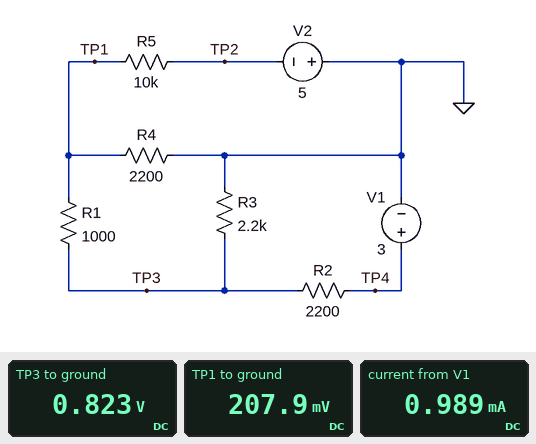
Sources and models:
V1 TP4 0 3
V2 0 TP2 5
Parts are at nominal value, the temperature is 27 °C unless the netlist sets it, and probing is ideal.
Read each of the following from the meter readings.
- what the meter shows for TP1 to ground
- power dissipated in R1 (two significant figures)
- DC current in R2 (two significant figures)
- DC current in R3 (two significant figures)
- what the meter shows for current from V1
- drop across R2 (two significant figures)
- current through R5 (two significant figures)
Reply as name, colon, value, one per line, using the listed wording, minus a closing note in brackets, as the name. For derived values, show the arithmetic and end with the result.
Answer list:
what the meter shows for TP1 to ground: 207.9 mV
power dissipated in R1: (823 mV - 207.9 mV)^2 / 1 kΩ = 380 µW
DC current in R2: (3 V - 823 mV) / 2.2 kΩ = 990 µA
DC current in R3: (823 mV) / 2.2 kΩ = 370 µA
what the meter shows for current from V1: 0.989 mA
drop across R2: 3 V - 823 mV = 2.2 V
current through R5: (207.9 mV - (-5 V)) / 10 kΩ = 520 µA
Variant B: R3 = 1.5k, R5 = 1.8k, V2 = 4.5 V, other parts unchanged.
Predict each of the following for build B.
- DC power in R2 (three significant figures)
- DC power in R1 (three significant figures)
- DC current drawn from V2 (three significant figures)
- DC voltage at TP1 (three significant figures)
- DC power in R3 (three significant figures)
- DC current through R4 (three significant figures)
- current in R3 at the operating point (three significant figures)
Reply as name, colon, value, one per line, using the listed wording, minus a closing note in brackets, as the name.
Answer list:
DC power in R2: 3.89 mW
DC power in R1: 1.64 mW
DC current drawn from V2: 1.83 mA
DC voltage at TP1: -1.21 V
DC power in R3: 3.64 µW
DC current through R4: 549 µA
current in R3 at the operating point: 49.2 µA
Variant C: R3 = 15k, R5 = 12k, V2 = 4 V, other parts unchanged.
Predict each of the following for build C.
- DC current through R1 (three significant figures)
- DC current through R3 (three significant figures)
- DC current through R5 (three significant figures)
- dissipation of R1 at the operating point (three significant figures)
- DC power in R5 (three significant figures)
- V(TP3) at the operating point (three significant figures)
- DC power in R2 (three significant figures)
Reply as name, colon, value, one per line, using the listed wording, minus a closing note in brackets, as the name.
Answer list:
DC current through R1: 677 µA
DC current through R3: 87.8 µA
DC current through R5: 387 µA
dissipation of R1 at the operating point: 459 µW
DC power in R5: 1.79 mW
V(TP3) at the operating point: 1.32 V
DC power in R2: 1.29 mW
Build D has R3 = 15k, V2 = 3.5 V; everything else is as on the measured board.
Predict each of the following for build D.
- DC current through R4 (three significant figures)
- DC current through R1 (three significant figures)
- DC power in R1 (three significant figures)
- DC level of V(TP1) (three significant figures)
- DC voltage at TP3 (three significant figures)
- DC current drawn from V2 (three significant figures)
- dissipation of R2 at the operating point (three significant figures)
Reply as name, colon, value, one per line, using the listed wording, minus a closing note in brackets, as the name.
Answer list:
DC current through R4: 277 µA
DC current through R1: 688 µA
DC power in R1: 473 µW
DC level of V(TP1): 609 mV
DC voltage at TP3: 1.30 V
DC current drawn from V2: 411 µA
dissipation of R2 at the operating point: 1.32 mW
